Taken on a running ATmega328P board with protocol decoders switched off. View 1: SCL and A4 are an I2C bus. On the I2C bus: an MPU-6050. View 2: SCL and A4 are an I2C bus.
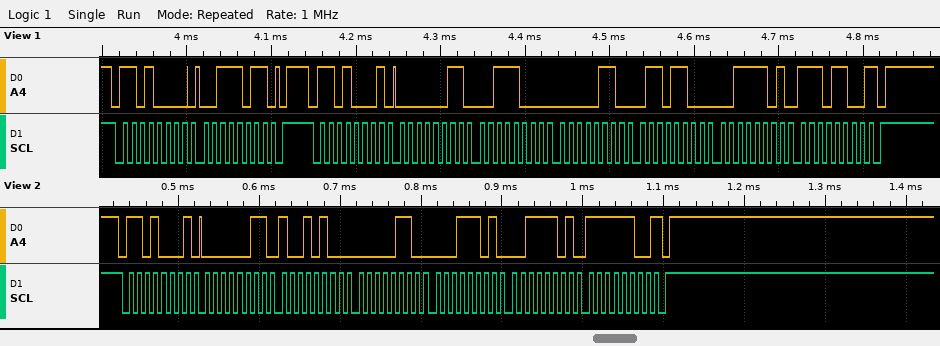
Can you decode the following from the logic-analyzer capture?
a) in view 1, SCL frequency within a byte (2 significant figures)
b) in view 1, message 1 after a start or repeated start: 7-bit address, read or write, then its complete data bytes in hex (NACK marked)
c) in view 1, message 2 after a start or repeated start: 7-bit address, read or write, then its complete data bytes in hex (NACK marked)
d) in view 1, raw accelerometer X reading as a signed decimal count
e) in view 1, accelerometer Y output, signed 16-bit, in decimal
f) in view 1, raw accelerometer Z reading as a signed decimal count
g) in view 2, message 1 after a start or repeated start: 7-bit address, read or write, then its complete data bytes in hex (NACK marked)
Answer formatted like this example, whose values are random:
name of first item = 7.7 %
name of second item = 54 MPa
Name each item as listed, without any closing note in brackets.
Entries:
in view 1, SCL frequency within a byte = 100 kHz
in view 1, message 1 after a start or repeated start: 7-bit address, read or write, then its complete data bytes in hex = 0x68 write: 3B
in view 1, message 2 after a start or repeated start: 7-bit address, read or write, then its complete data bytes in hex = 0x68 read: 03 38 06 6C 3D EC NACK
in view 1, raw accelerometer X reading as a signed decimal count = 824
in view 1, accelerometer Y output, signed 16-bit, in decimal = 1644
in view 1, raw accelerometer Z reading as a signed decimal count = 15852
in view 2, message 1 after a start or repeated start: 7-bit address, read or write, then its complete data bytes in hex = 0x68 read: 03 94 06 1D 3D FC NACK
